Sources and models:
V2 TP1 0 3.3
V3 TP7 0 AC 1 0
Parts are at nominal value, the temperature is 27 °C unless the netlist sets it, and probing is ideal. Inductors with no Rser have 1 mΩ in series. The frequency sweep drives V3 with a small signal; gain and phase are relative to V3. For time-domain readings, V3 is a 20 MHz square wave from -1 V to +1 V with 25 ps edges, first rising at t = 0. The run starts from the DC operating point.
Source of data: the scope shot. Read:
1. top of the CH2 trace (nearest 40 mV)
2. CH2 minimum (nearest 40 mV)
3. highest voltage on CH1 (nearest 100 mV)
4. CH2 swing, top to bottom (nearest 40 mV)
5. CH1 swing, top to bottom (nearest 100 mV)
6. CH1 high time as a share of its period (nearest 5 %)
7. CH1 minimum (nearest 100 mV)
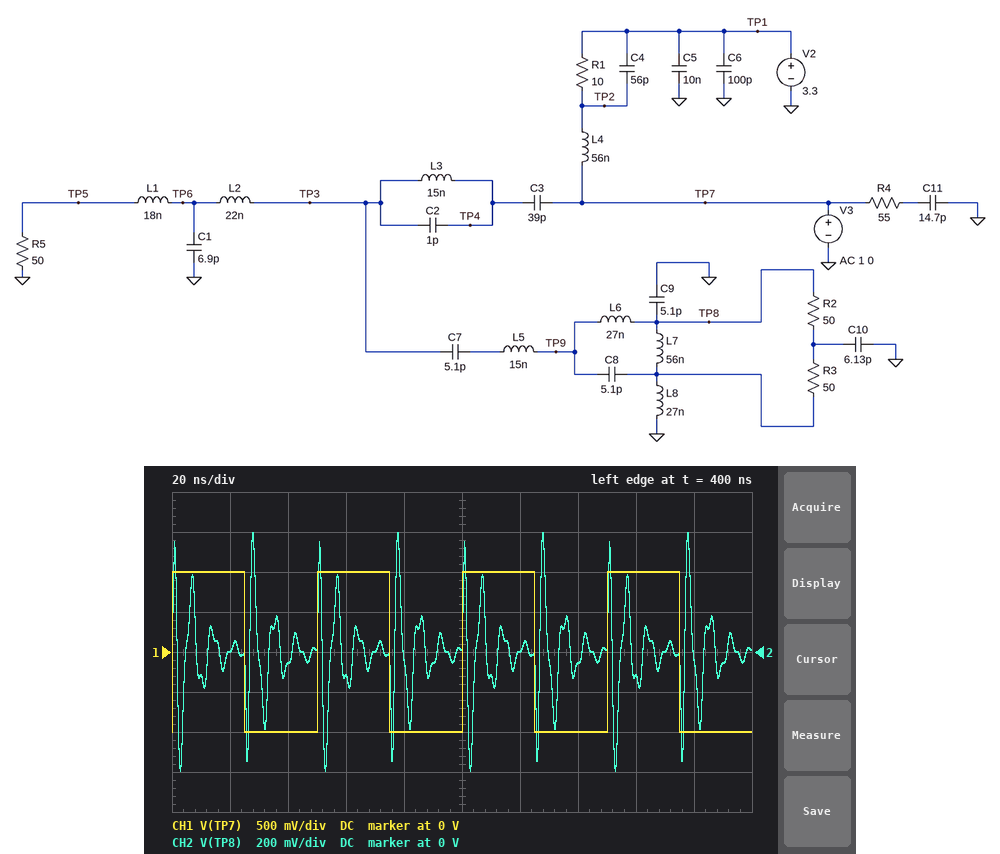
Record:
600 mV
-600 mV
1.0 V
1.20 V
2.0 V
50 %
-1.0 V
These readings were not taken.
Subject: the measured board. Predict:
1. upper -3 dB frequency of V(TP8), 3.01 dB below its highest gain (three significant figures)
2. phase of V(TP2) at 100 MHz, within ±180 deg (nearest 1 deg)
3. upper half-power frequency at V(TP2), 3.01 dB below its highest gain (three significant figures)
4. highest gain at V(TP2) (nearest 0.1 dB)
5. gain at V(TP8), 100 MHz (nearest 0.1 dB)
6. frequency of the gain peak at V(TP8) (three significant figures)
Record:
360 MHz
-94 deg
31.5 MHz
0 dB
-10.5 dB
342 MHz
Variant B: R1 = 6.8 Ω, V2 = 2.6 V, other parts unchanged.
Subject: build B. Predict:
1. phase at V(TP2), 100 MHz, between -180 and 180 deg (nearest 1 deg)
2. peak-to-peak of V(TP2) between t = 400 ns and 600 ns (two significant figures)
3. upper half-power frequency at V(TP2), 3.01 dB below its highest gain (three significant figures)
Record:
-93 deg
1.8 V
20.3 MHz
